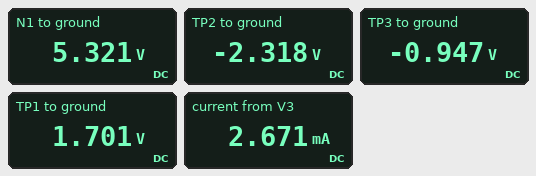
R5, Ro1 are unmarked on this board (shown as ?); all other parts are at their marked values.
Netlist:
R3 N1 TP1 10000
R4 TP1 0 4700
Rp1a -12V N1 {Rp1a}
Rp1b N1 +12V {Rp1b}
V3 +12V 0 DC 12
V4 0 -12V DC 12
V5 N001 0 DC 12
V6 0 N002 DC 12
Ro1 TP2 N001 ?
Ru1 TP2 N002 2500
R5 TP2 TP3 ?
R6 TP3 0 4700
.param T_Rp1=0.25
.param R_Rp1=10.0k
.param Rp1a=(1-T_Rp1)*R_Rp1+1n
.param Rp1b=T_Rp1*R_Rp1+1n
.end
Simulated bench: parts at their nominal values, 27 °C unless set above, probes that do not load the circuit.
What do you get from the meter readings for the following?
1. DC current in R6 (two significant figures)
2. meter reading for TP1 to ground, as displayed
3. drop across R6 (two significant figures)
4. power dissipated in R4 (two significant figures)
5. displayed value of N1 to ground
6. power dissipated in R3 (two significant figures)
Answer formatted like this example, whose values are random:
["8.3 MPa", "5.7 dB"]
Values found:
["200 µA", "1.701 V", "950 mV", "620 µW", "5.321 V", "1.3 mW"]
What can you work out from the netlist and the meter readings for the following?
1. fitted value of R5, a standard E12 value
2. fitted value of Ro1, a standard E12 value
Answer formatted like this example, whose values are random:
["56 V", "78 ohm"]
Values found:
["6.8 kΩ", "3.9 kΩ"]
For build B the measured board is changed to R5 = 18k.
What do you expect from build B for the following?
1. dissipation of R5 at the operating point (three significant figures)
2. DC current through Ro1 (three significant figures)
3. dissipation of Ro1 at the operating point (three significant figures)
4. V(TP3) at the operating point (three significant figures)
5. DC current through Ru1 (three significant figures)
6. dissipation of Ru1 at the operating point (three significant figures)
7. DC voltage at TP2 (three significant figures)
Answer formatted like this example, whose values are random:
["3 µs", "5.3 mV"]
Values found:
["211 µW", "3.71 mA", "53.6 mW", "-509 mV", "3.82 mA", "36.4 mW", "-2.46 V"]
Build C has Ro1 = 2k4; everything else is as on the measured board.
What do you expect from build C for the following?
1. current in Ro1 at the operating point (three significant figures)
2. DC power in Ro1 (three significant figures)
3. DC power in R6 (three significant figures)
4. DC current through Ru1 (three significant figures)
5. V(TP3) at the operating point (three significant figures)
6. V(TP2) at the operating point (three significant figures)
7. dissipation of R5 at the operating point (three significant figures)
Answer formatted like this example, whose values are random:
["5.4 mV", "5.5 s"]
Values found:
["4.91 mA", "57.8 mW", "1.74 µW", "4.89 mA", "90.5 mV", "221 mV", "2.52 µW"]
